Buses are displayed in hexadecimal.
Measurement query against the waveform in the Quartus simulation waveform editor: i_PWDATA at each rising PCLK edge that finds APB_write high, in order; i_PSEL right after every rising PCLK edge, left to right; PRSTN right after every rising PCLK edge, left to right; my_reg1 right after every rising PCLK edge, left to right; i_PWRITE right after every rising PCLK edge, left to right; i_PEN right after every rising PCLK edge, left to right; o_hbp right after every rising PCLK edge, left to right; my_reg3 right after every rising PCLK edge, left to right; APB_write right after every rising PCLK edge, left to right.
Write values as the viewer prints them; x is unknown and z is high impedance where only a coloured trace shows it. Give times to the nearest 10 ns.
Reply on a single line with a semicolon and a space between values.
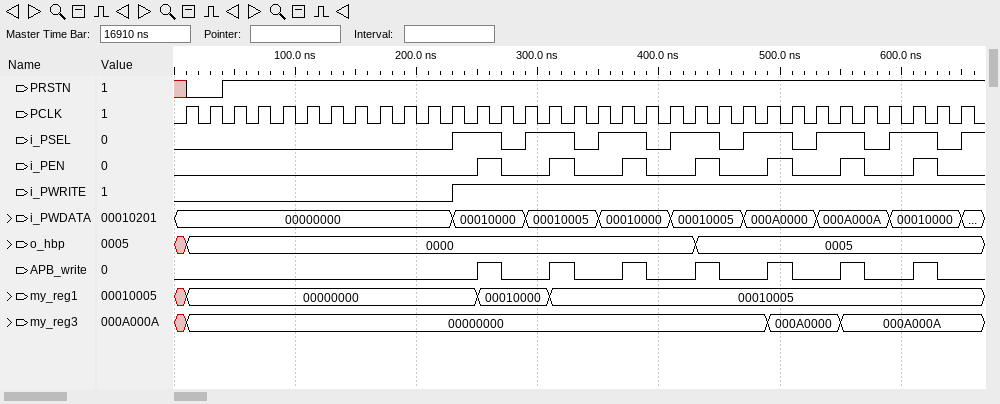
00010000, 00010005, 00010000, 00010005, 000A0000, 000A000A, 00010000; 0 0 0 0 0 0 0 0 0 0 0 1 1 0 1 1 0 1 1 0 1 1 0 1 1 0 1 1 0 1 1 0 1; 0 0 1 1 1 1 1 1 1 1 1 1 1 1 1 1 1 1 1 1 1 1 1 1 1 1 1 1 1 1 1 1 1; 00000000, 00000000, 00000000, 00000000, 00000000, 00000000, 00000000, 00000000, 00000000, 00000000, 00000000, 00000000, 00010000, 00010000, 00010000, 00010005, 00010005, 00010005, 00010005, 00010005, 00010005, 00010005, 00010005, 00010005, 00010005, 00010005, 00010005, 00010005, 00010005, 00010005, 00010005, 00010005, 00010005; 0 0 0 0 0 0 0 0 0 0 0 1 1 1 1 1 1 1 1 1 1 1 1 1 1 1 1 1 1 1 1 1 1; 0 0 0 0 0 0 0 0 0 0 0 0 1 0 0 1 0 0 1 0 0 1 0 0 1 0 0 1 0 0 1 0 0; 0000, 0000, 0000, 0000, 0000, 0000, 0000, 0000, 0000, 0000, 0000, 0000, 0000, 0000, 0000, 0000, 0000, 0000, 0000, 0000, 0000, 0005, 0005, 0005, 0005, 0005, 0005, 0005, 0005, 0005, 0005, 0005, 0005; 00000000, 00000000, 00000000, 00000000, 00000000, 00000000, 00000000, 00000000, 00000000, 00000000, 00000000, 00000000, 00000000, 00000000, 00000000, 00000000, 00000000, 00000000, 00000000, 00000000, 00000000, 00000000, 00000000, 00000000, 000A0000, 000A0000, 000A0000, 000A000A, 000A000A, 000A000A, 000A000A, 000A000A, 000A000A; 0 0 0 0 0 0 0 0 0 0 0 0 1 0 0 1 0 0 1 0 0 1 0 0 1 0 0 1 0 0 1 0 0
